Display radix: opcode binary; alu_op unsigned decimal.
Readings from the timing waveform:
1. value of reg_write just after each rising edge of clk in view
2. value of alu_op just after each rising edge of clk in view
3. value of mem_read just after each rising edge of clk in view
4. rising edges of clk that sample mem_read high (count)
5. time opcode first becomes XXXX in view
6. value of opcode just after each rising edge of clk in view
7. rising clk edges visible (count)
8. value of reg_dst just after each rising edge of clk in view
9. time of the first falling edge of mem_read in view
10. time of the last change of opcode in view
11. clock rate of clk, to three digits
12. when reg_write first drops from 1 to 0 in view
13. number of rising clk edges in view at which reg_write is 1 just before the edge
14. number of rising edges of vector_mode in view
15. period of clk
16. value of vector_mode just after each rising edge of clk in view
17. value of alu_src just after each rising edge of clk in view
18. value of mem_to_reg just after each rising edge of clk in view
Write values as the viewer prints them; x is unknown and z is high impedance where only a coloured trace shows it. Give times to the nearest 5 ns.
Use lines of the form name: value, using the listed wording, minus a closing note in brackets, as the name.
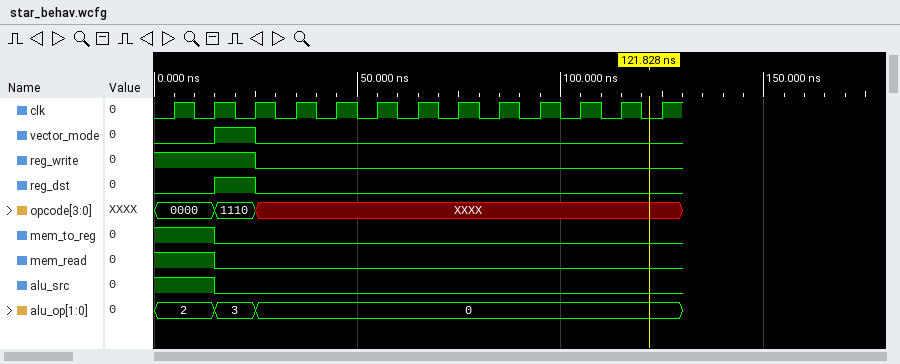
value of reg_write just after each rising edge of clk in view: 1 1 0 0 0 0 0 0 0 0 0 0 0
value of alu_op just after each rising edge of clk in view: 2, 3, 0, 0, 0, 0, 0, 0, 0, 0, 0, 0, 0
value of mem_read just after each rising edge of clk in view: 1 0 0 0 0 0 0 0 0 0 0 0 0
rising edges of clk that sample mem_read high: 2
time opcode first becomes XXXX in view: 25 ns
value of opcode just after each rising edge of clk in view: 0000, 1110, XXXX, XXXX, XXXX, XXXX, XXXX, XXXX, XXXX, XXXX, XXXX, XXXX, XXXX
rising clk edges visible: 13
value of reg_dst just after each rising edge of clk in view: 0 1 0 0 0 0 0 0 0 0 0 0 0
time of the first falling edge of mem_read in view: 15 ns
time of the last change of opcode in view: 25 ns
clock rate of clk, to three digits: 100 MHz
when reg_write first drops from 1 to 0 in view: 25 ns
number of rising clk edges in view at which reg_write is 1 just before the edge: 3
number of rising edges of vector_mode in view: 1
period of clk: 10 ns
value of vector_mode just after each rising edge of clk in view: 0 1 0 0 0 0 0 0 0 0 0 0 0
value of alu_src just after each rising edge of clk in view: 1 0 0 0 0 0 0 0 0 0 0 0 0
value of mem_to_reg just after each rising edge of clk in view: 1 0 0 0 0 0 0 0 0 0 0 0 0
